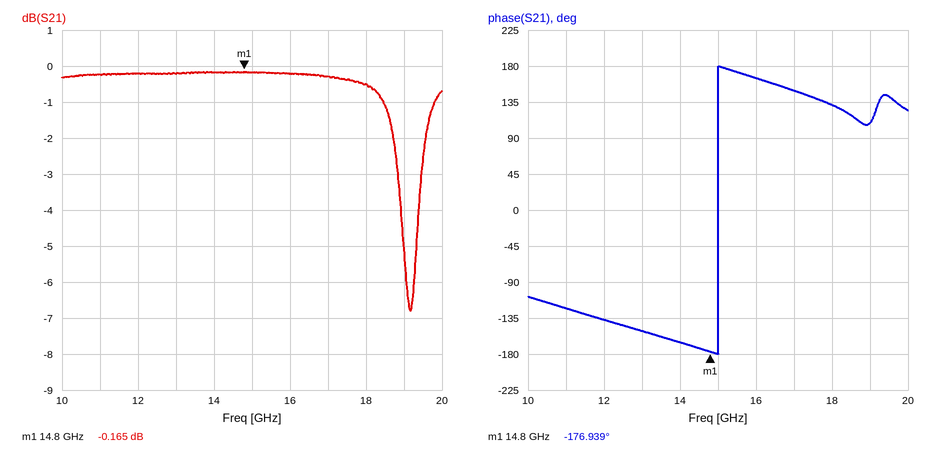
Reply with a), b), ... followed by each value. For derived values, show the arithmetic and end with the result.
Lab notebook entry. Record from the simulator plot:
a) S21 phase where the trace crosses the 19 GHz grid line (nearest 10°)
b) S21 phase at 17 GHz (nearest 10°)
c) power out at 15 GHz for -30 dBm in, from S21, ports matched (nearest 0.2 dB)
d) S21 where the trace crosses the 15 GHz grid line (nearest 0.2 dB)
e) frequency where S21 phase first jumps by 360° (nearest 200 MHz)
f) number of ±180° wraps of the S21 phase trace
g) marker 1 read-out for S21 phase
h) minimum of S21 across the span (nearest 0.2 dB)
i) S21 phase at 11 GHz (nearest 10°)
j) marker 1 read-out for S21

a) 110°
b) 150°
c) -30 dBm + (-0.2 dB) = -30.2 dBm
d) -0.2 dB
e) 15.0 GHz
f) 1
g) -176.939°
h) -6.8 dB
i) -120°
j) -0.165 dB
